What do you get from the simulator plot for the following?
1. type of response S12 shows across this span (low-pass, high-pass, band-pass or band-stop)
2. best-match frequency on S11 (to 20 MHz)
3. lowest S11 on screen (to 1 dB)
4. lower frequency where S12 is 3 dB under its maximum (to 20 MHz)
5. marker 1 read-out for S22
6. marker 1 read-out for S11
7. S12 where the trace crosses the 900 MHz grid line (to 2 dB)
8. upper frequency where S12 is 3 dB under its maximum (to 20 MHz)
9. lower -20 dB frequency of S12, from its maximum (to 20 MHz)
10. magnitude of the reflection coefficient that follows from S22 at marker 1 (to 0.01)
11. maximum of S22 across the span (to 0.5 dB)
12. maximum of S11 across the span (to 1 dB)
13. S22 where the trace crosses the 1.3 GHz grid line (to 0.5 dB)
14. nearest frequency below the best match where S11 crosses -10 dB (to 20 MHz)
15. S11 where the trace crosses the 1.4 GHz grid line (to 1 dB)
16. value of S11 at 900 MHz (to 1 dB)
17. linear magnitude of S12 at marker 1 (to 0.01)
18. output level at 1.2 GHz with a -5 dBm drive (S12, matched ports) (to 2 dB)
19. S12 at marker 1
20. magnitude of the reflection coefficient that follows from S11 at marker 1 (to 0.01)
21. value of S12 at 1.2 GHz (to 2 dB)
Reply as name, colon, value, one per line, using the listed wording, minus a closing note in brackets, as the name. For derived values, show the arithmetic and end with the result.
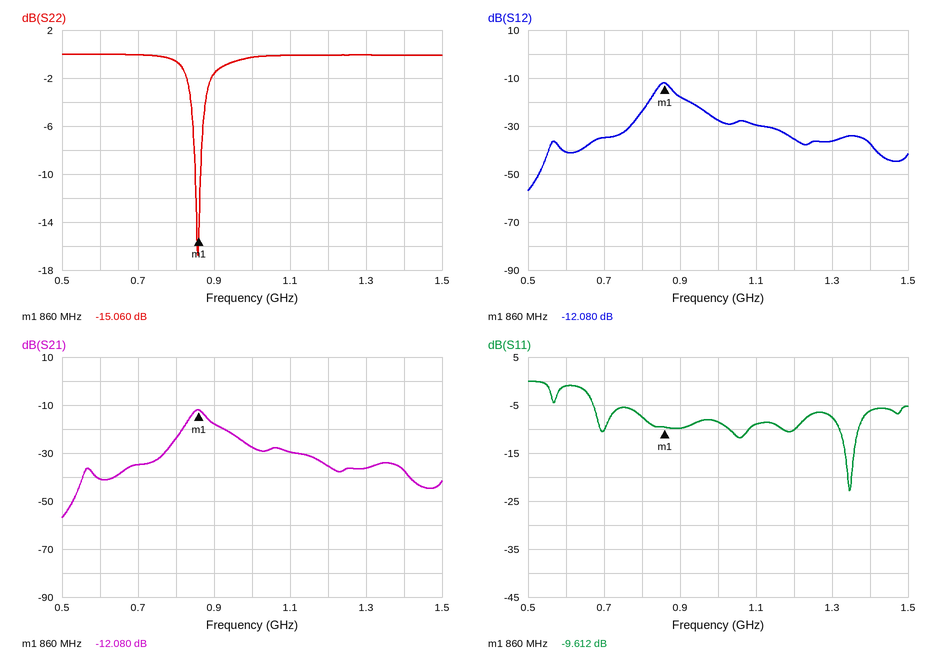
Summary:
type of response S12 shows across this span: band-pass
best-match frequency on S11: 1.34 GHz
lowest S11 on screen: -23 dB
lower frequency where S12 is 3 dB under its maximum: 840 MHz
marker 1 read-out for S22: -15.060 dB
marker 1 read-out for S11: -9.612 dB
S12 where the trace crosses the 900 MHz grid line: -18 dB
upper frequency where S12 is 3 dB under its maximum: 880 MHz
lower -20 dB frequency of S12, from its maximum: 760 MHz
magnitude of the reflection coefficient that follows from S22 at marker 1: 10^(-15.06/20) ≈ 0.18
maximum of S22 across the span: 0.0 dB
maximum of S11 across the span: 0 dB
S22 where the trace crosses the 1.3 GHz grid line: 0.0 dB
nearest frequency below the best match where S11 crosses -10 dB: 1.32 GHz
S11 where the trace crosses the 1.4 GHz grid line: -6 dB
value of S11 at 900 MHz: -10 dB
linear magnitude of S12 at marker 1: 10^(-12.08/20) ≈ 0.25
output level at 1.2 GHz with a -5 dBm drive (S12, matched ports): -5 dBm + (-36 dB) = -40 dBm
S12 at marker 1: -12.080 dB
magnitude of the reflection coefficient that follows from S11 at marker 1: 10^(-9.612/20) ≈ 0.33
value of S12 at 1.2 GHz: -36 dB
